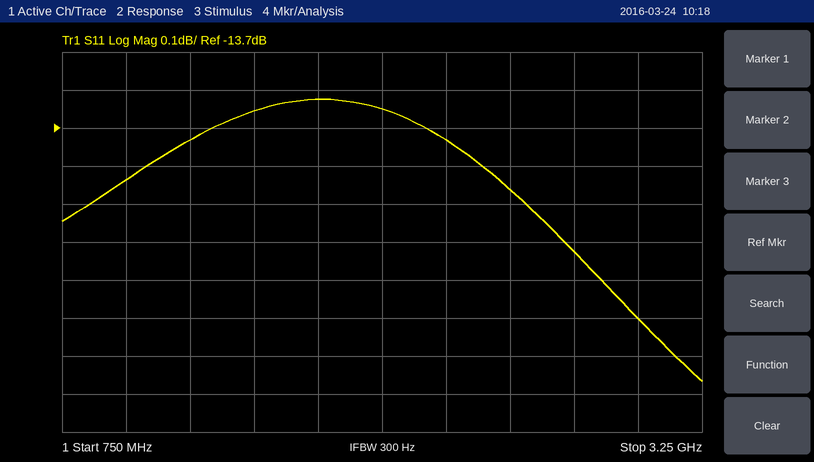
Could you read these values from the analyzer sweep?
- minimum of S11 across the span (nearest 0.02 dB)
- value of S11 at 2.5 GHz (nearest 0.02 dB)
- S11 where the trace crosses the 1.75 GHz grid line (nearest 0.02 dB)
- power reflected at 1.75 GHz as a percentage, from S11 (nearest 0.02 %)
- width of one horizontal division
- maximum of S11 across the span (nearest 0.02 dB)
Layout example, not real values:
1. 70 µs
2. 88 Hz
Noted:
1. -14.36 dB
2. -13.86 dB
3. -13.62 dB
4. 4.34 %
5. 250 MHz
6. -13.62 dB
